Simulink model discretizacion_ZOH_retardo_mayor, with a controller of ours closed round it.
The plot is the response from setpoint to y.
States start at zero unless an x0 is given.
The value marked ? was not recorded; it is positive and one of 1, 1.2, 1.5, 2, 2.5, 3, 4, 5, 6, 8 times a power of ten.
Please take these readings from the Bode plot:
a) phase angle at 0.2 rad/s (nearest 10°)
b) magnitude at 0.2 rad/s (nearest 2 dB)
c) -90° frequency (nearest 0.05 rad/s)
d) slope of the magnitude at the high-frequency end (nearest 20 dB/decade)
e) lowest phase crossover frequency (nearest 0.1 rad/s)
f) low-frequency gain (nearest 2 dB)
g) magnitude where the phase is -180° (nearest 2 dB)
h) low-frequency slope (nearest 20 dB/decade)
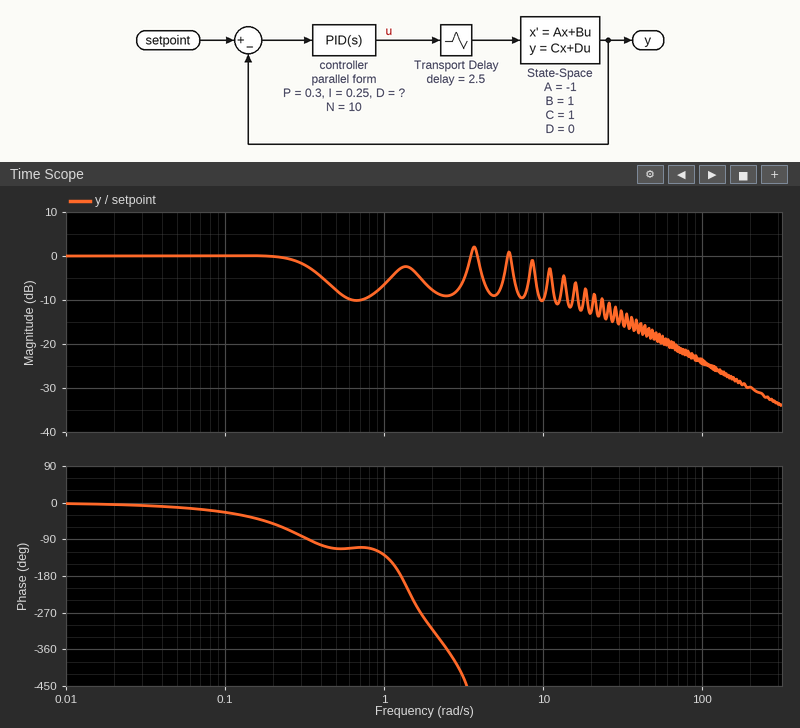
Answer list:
-50°
0 dB
0.35 rad/s
-20 dB/decade
1.3 rad/s
0 dB
-2 dB
0 dB/decade
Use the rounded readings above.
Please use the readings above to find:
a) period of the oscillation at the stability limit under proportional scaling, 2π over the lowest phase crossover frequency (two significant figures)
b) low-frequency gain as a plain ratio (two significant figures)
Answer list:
4.8 s
1.0
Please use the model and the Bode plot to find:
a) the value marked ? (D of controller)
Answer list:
0.6
